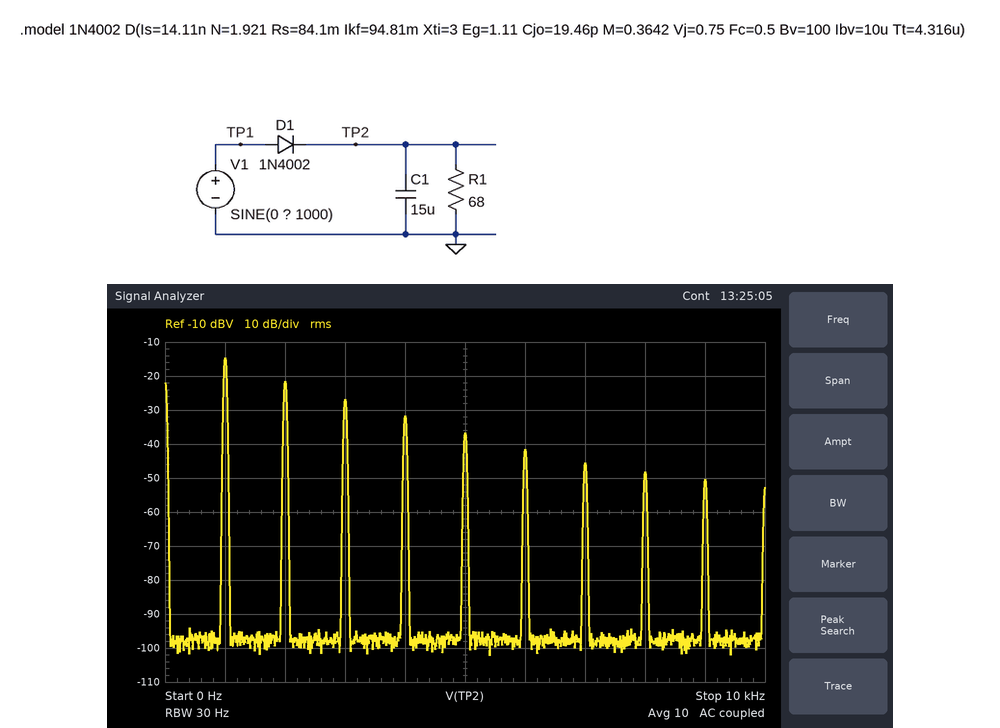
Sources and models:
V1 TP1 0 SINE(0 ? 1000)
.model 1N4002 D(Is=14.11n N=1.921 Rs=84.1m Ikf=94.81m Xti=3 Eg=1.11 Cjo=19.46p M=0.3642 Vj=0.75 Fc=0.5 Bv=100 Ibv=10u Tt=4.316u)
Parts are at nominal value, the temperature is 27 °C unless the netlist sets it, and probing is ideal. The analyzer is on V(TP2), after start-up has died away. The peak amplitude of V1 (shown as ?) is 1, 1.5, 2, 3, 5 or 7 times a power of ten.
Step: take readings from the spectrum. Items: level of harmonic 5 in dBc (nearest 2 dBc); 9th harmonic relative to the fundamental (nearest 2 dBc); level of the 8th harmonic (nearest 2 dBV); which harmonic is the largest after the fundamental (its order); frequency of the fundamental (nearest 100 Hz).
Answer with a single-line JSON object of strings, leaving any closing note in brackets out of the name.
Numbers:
{"level of harmonic 5 in dBc": "-22 dBc", "9th harmonic relative to the fundamental": "-36 dBc", "level of the 8th harmonic": "-48 dBV", "which harmonic is the largest after the fundamental": "2", "frequency of the fundamental": "1.0 kHz"}
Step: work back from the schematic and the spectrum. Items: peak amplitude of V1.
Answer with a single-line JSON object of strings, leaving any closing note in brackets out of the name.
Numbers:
{"peak amplitude of V1": "2 V"}
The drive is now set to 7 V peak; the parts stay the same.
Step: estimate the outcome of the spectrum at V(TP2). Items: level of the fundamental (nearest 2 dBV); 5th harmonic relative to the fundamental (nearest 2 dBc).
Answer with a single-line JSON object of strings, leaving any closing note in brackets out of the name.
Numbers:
{"level of the fundamental": "0 dBV", "5th harmonic relative to the fundamental": "-24 dBc"}
